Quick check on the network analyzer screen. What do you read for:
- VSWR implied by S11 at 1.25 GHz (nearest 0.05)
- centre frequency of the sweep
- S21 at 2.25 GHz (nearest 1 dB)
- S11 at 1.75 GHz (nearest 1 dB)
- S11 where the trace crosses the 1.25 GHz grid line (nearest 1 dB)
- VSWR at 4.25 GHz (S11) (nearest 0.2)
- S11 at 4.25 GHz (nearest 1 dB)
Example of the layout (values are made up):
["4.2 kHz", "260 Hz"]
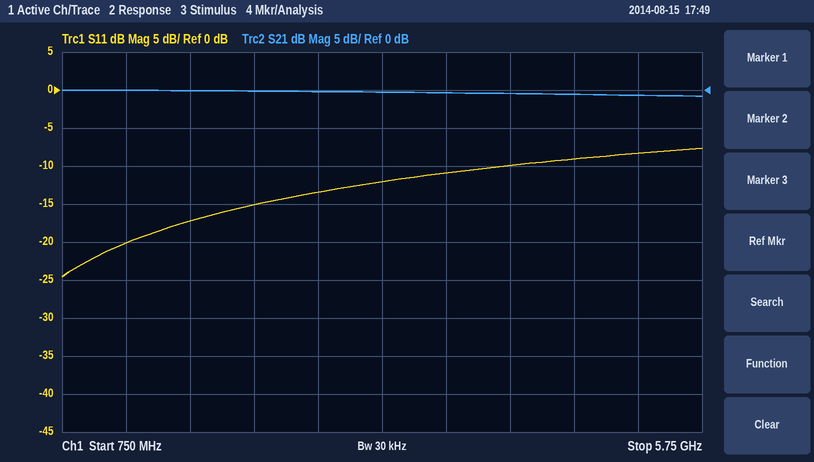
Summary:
["1.20", "3.25 GHz", "0 dB", "-17 dB", "-20 dB", "2.0", "-10 dB"]
